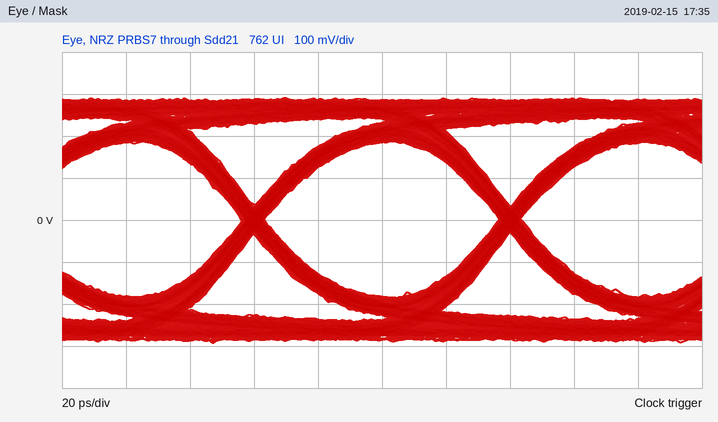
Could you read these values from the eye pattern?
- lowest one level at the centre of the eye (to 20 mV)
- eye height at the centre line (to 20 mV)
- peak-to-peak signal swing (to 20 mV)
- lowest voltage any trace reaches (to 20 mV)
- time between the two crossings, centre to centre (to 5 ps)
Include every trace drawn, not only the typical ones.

180 mV
360 mV
580 mV
-300 mV
80 ps
